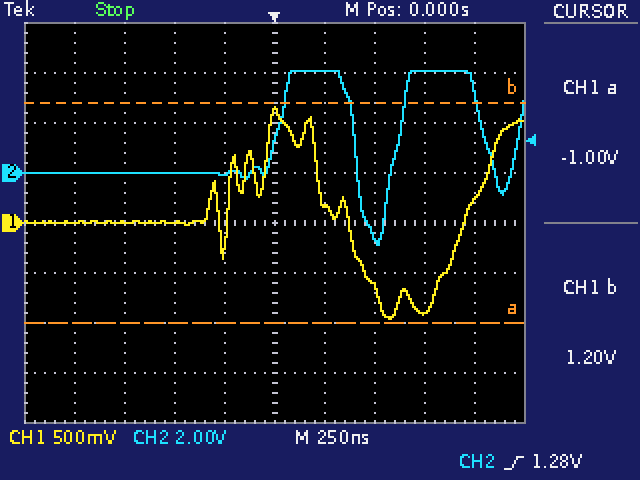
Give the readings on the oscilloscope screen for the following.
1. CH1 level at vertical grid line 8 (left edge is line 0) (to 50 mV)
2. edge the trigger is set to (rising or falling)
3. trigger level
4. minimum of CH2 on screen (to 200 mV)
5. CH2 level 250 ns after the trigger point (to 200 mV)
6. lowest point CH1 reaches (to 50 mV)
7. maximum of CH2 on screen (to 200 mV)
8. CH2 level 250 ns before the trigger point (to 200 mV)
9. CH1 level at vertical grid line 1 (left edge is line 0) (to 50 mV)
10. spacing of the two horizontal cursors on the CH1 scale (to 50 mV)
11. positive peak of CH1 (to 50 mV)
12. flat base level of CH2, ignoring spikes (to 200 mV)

-900 mV
rising
1.28 V
-2.8 V
4.0 V
-950 mV
4.0 V
0.0 V
0 mV
2.20 V
1.15 V
0.0 V
